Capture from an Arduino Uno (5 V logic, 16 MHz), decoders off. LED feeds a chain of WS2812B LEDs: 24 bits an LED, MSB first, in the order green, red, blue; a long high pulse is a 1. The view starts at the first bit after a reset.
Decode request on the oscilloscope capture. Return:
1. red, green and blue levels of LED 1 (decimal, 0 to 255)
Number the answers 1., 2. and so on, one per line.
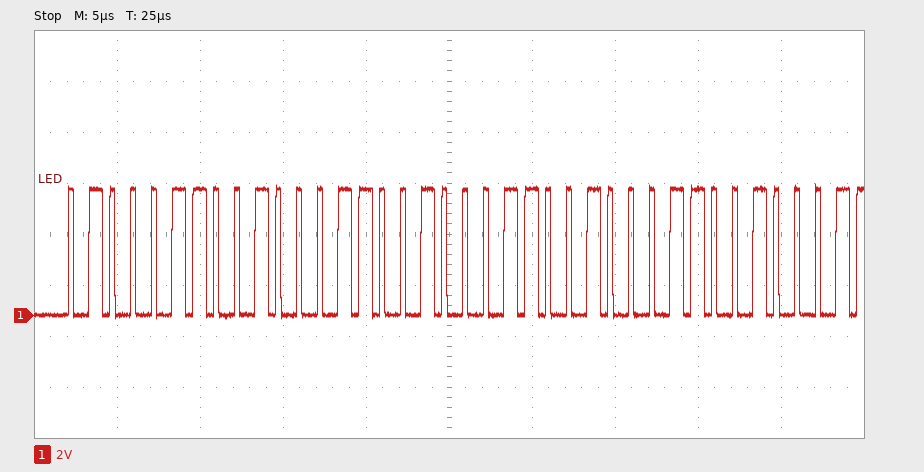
1. 70, 70, 70
